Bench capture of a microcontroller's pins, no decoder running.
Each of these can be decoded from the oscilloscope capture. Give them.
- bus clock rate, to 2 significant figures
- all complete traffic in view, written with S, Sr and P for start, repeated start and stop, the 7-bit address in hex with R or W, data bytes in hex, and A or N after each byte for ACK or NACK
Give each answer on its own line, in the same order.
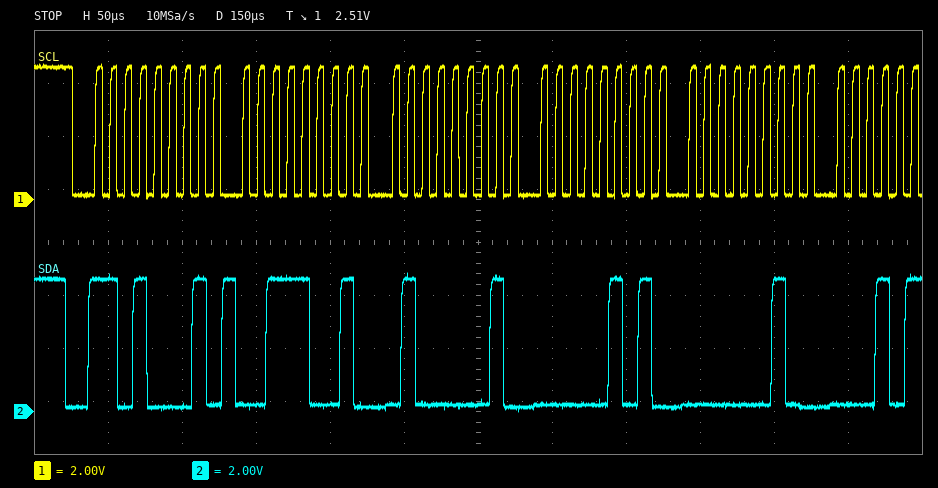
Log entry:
100 kHz
S 68R A 39 A 41 A 05 A 02 A
